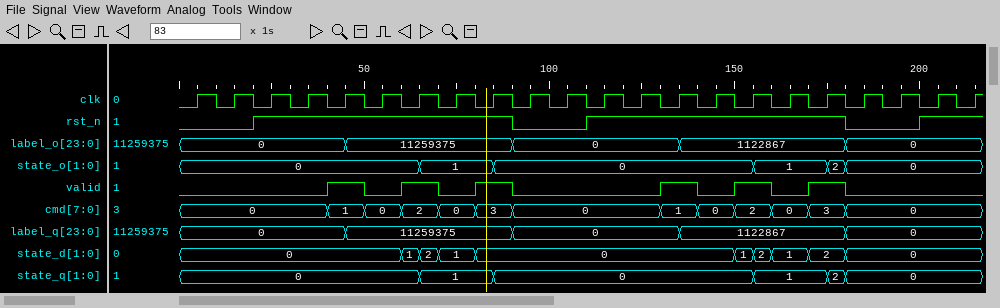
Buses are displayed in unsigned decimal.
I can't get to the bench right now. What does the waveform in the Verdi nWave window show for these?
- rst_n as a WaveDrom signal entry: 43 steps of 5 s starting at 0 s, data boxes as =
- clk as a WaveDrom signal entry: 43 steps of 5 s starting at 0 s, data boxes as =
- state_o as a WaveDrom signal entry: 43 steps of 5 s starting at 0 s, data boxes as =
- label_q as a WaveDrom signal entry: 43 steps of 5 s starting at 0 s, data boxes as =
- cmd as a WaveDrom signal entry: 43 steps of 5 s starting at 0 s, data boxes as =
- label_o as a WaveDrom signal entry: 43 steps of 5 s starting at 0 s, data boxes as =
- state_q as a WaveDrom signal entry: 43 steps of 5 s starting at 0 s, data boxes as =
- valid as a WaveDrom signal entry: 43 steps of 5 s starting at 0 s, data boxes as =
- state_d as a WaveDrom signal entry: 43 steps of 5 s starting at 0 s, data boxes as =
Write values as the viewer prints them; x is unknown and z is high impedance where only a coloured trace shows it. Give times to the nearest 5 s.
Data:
{name: 'rst_n', wave: '0...1.............0...1.............0...1..'}
{name: 'clk', wave: '0101010101010101010101010101010101010101010'}
{name: 'state_o', wave: '=............=...=.............=...==......', data: '0 1 0 1 2 0'}
{name: 'label_q', wave: '=........=........=........=........=......', data: '0 11259375 0 1122867 0'}
{name: 'cmd', wave: '=.......=.=.=.=.=.=.......=.=.=.=.=.=......', data: '0 1 0 2 0 3 0 1 0 2 0 3 0'}
{name: 'label_o', wave: '=........=........=........=........=......', data: '0 11259375 0 1122867 0'}
{name: 'state_q', wave: '=............=...=.............=...==......', data: '0 1 0 1 2 0'}
{name: 'valid', wave: '0.......1.0.1.0.1.0.......1.0.1.0.1.0......'}
{name: 'state_d', wave: '=...........===.=.............===.=.=......', data: '0 1 2 1 0 1 2 1 2 0'}
